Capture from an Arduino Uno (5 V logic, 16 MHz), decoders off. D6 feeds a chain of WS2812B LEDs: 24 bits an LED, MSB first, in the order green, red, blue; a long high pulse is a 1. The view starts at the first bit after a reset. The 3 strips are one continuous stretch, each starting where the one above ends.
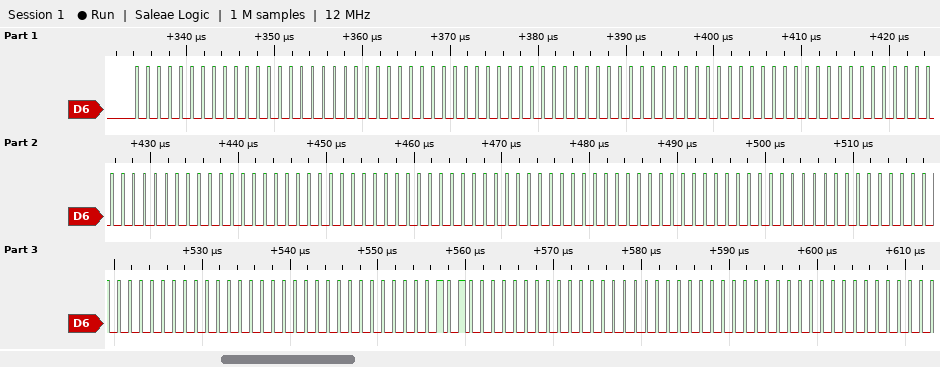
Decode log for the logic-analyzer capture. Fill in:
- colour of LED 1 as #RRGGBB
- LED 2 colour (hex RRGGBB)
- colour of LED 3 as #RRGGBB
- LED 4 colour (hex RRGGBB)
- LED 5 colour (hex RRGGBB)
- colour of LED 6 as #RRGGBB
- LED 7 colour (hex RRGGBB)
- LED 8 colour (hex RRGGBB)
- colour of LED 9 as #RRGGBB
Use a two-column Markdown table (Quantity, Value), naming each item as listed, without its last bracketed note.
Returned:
| Quantity | Value |
|---|---|
| colour of LED 1 as #RRGGBB | #000000 |
| LED 2 colour | #000000 |
| colour of LED 3 as #RRGGBB | #000000 |
| LED 4 colour | #000000 |
| LED 5 colour | #000000 |
| colour of LED 6 as #RRGGBB | #000000 |
| LED 7 colour | #000000 |
| LED 8 colour | #280000 |
| colour of LED 9 as #RRGGBB | #000000 |
